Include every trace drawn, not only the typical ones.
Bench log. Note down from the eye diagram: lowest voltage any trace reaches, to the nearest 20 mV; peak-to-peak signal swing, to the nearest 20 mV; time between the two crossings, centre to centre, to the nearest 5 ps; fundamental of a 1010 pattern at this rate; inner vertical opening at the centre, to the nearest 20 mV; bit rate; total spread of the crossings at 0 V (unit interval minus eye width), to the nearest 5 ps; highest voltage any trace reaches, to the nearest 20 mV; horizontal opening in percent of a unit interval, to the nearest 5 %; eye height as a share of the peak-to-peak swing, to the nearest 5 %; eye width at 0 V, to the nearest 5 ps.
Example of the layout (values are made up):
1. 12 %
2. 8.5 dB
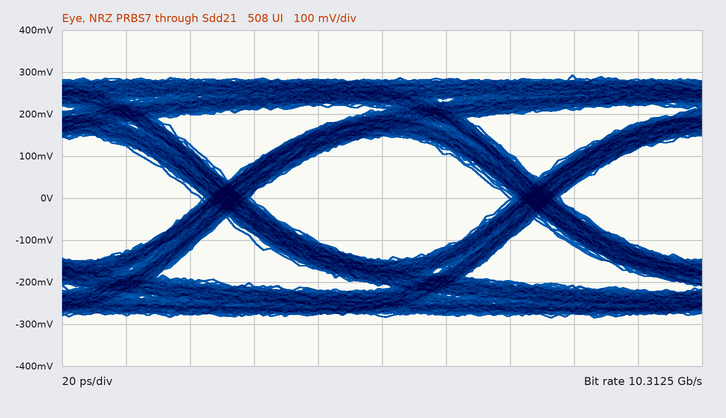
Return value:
1. -280 mV
2. 580 mV
3. 95 ps
4. 5.15625 GHz
5. 300 mV
6. 10.3125 Gb/s
7. 15 ps
8. 300 mV
9. 85 %
10. 50 %
11. 80 ps
